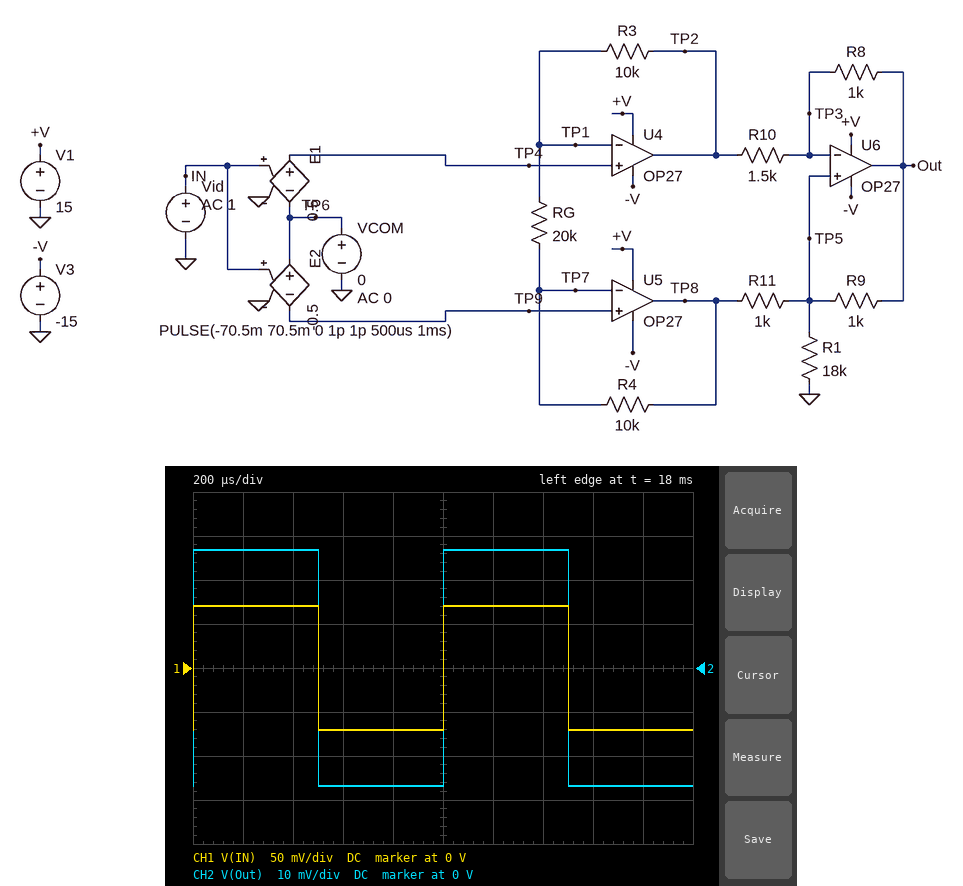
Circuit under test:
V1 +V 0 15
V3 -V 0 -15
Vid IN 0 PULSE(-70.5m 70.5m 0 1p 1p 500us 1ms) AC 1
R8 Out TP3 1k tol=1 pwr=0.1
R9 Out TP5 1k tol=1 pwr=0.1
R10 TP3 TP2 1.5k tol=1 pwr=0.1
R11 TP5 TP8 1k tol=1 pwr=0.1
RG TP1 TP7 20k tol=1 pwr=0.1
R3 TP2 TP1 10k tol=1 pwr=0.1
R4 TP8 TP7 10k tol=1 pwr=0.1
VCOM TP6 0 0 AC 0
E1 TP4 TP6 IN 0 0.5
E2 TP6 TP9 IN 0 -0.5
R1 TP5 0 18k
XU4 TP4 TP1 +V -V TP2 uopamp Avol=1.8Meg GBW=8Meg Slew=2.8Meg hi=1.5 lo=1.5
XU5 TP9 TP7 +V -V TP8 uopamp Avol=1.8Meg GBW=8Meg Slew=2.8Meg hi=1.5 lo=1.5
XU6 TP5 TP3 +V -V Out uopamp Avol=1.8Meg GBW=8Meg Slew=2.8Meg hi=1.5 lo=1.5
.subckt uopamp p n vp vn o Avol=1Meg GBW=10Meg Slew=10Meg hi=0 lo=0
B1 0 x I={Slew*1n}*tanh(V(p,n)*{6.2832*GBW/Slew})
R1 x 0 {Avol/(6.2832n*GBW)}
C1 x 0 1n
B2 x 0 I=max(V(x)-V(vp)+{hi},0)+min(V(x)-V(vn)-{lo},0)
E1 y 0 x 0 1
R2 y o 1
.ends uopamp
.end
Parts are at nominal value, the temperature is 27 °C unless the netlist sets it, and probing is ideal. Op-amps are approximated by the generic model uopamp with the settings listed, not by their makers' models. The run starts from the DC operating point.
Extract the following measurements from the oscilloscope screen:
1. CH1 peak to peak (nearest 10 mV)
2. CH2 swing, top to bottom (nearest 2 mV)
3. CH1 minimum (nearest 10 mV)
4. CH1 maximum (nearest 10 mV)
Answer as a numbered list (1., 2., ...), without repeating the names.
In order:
1. 140 mV
2. 54 mV
3. -70 mV
4. 70 mV
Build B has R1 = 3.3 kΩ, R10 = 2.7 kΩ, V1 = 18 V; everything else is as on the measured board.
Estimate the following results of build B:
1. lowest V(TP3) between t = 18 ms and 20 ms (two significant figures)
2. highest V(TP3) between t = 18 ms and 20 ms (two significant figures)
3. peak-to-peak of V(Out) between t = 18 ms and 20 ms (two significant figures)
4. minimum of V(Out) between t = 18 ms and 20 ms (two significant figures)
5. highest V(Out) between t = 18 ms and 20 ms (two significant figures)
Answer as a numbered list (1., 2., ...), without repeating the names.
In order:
1. -24 mV
2. 24 mV
3. 39 mV
4. -20 mV
5. 20 mV
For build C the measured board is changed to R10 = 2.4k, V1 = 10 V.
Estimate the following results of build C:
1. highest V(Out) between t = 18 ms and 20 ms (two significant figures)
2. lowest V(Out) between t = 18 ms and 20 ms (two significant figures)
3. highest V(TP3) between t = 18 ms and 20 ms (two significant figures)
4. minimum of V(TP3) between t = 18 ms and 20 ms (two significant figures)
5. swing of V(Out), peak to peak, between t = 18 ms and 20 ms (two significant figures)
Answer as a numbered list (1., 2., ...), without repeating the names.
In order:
1. 31 mV
2. -31 mV
3. 32 mV
4. -32 mV
5. 62 mV
